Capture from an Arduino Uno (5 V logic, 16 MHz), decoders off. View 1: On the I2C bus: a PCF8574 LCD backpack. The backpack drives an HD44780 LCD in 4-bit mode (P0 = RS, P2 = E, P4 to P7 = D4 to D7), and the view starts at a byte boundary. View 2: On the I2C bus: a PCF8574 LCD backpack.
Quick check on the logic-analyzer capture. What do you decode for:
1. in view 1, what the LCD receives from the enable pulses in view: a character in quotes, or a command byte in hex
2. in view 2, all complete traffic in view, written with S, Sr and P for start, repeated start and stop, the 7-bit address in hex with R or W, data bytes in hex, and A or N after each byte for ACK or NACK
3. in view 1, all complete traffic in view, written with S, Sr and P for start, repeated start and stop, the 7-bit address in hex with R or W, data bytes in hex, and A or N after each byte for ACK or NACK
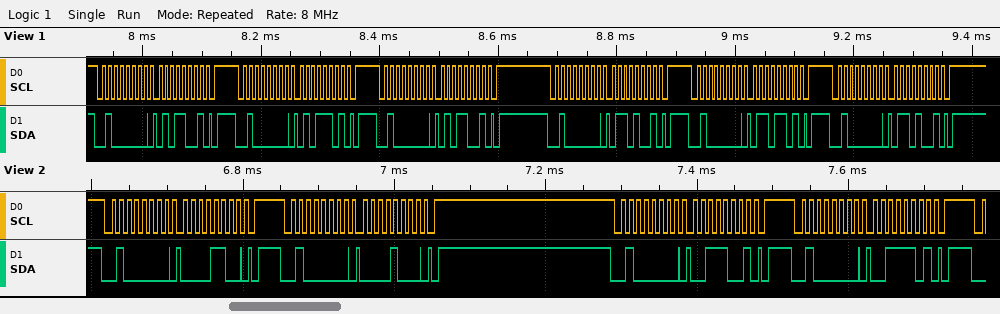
'V'
S 20W A 0C A P S 20W A 08 A P S 20W A 39 A P S 20W A 3D A P
S 20W A 59 A P S 20W A 5D A P S 20W A 59 A P S 20W A 69 A P S 20W A 6D A P S 20W A 69 A P
